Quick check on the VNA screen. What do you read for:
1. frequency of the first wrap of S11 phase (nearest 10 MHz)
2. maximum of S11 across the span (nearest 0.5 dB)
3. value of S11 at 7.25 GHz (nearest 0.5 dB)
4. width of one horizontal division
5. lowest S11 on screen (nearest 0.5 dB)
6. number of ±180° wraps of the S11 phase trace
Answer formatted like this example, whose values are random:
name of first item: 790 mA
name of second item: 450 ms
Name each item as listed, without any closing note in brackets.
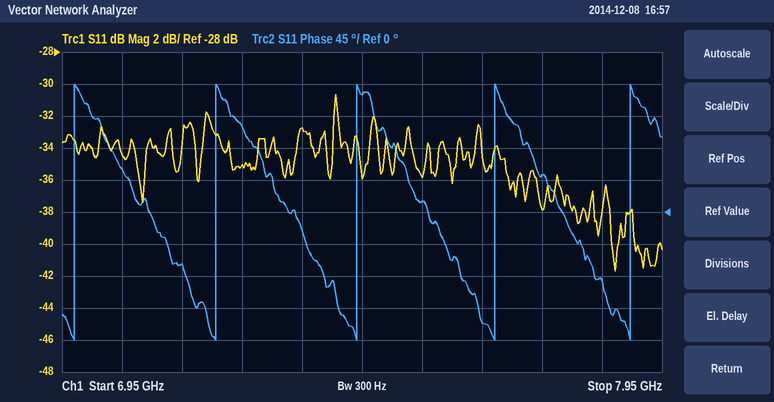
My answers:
frequency of the first wrap of S11 phase: 6.97 GHz
maximum of S11 across the span: -30.5 dB
value of S11 at 7.25 GHz: -35.0 dB
width of one horizontal division: 100 MHz
lowest S11 on screen: -41.5 dB
number of ±180° wraps of the S11 phase trace: 5
